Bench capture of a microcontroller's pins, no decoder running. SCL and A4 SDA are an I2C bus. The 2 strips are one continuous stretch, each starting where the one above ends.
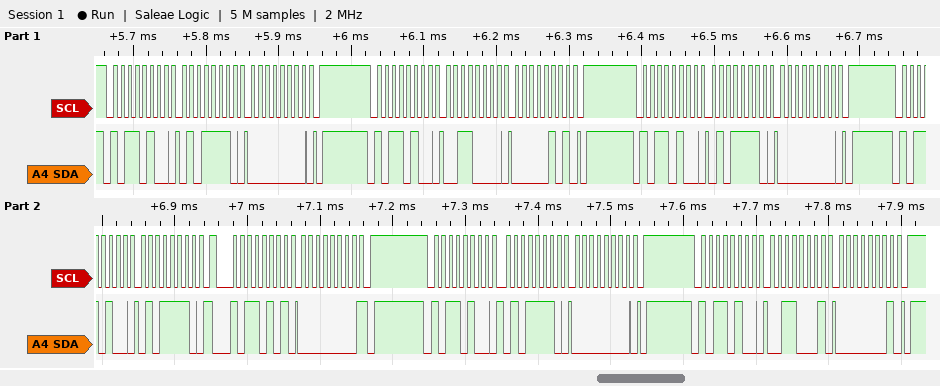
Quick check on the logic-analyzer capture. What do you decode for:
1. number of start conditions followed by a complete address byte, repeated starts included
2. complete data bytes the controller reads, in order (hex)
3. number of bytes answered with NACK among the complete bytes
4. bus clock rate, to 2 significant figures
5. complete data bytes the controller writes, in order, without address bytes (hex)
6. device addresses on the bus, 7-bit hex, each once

7
00
1
100 kHz
5E 00 30 05 5E 00 5E 5E 00 31 01
0x5A
